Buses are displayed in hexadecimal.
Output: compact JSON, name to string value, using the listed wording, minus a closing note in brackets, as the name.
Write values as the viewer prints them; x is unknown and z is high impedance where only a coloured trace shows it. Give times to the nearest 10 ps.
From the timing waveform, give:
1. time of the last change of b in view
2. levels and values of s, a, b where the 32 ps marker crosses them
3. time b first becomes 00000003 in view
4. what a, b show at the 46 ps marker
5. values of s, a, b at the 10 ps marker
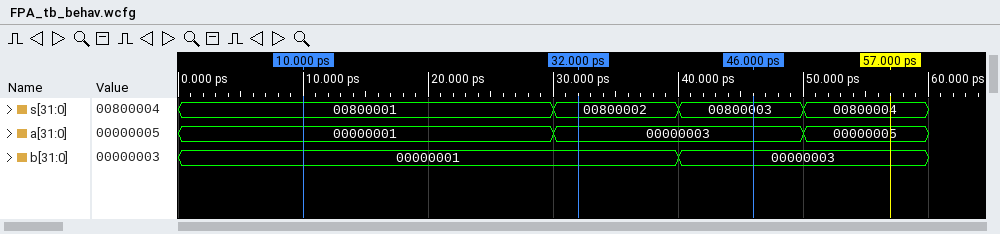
{"time of the last change of b in view": "40 ps", "levels and values of s, a, b where the 32 ps marker crosses them": "s=00800002, a=00000003, b=00000001", "time b first becomes 00000003 in view": "40 ps", "what a, b show at the 46 ps marker": "a=00000003, b=00000003", "values of s, a, b at the 10 ps marker": "s=00800001, a=00000001, b=00000001"}
